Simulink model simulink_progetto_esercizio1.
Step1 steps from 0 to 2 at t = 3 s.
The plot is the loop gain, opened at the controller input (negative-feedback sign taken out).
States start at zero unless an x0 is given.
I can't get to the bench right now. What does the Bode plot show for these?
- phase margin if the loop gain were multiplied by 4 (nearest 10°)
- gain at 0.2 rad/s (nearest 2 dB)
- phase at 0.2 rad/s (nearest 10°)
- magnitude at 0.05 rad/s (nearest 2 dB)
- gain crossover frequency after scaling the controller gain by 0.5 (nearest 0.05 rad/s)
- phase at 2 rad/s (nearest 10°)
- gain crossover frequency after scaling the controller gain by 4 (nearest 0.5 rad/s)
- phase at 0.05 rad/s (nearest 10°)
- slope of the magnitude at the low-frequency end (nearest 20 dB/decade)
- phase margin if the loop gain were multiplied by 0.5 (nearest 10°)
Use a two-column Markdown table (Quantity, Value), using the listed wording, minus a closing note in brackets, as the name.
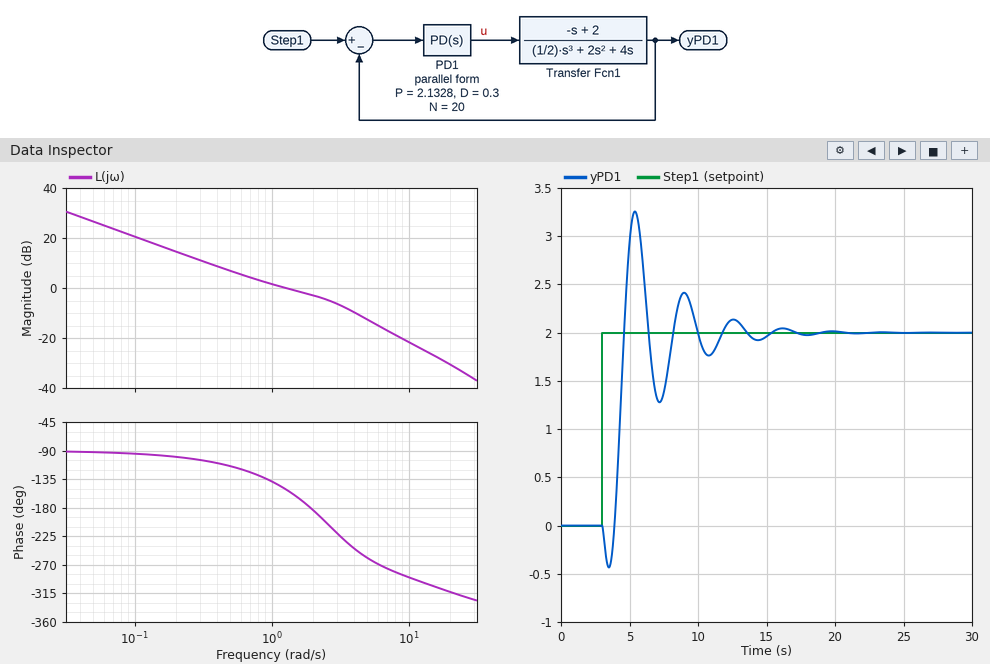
| Quantity | Value |
|---|---|
| phase margin if the loop gain were multiplied by 4 | -80° |
| gain at 0.2 rad/s | 14 dB |
| phase at 0.2 rad/s | -100° |
| magnitude at 0.05 rad/s | 26 dB |
| gain crossover frequency after scaling the controller gain by 0.5 | 0.55 rad/s |
| phase at 2 rad/s | -180° |
| gain crossover frequency after scaling the controller gain by 4 | 5.0 rad/s |
| phase at 0.05 rad/s | -90° |
| slope of the magnitude at the low-frequency end | -20 dB/decade |
| phase margin if the loop gain were multiplied by 0.5 | 60° |
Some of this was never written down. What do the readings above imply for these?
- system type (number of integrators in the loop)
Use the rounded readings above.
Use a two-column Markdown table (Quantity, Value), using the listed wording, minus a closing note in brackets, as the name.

| Quantity | Value |
|---|---|
| system type | 1 |
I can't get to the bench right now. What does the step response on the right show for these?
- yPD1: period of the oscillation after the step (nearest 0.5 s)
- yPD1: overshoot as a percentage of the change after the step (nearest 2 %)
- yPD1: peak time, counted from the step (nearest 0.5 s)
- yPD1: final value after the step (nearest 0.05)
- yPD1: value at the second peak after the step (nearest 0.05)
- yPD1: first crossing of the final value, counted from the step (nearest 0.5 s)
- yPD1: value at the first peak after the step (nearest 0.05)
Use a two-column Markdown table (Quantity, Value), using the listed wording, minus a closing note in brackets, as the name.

| Quantity | Value |
|---|---|
| yPD1: period of the oscillation after the step | 3.5 s |
| yPD1: overshoot as a percentage of the change after the step | 62 % |
| yPD1: peak time, counted from the step | 2.5 s |
| yPD1: final value after the step | 2.00 |
| yPD1: value at the second peak after the step | 2.40 |
| yPD1: first crossing of the final value, counted from the step | 1.5 s |
| yPD1: value at the first peak after the step | 3.25 |
